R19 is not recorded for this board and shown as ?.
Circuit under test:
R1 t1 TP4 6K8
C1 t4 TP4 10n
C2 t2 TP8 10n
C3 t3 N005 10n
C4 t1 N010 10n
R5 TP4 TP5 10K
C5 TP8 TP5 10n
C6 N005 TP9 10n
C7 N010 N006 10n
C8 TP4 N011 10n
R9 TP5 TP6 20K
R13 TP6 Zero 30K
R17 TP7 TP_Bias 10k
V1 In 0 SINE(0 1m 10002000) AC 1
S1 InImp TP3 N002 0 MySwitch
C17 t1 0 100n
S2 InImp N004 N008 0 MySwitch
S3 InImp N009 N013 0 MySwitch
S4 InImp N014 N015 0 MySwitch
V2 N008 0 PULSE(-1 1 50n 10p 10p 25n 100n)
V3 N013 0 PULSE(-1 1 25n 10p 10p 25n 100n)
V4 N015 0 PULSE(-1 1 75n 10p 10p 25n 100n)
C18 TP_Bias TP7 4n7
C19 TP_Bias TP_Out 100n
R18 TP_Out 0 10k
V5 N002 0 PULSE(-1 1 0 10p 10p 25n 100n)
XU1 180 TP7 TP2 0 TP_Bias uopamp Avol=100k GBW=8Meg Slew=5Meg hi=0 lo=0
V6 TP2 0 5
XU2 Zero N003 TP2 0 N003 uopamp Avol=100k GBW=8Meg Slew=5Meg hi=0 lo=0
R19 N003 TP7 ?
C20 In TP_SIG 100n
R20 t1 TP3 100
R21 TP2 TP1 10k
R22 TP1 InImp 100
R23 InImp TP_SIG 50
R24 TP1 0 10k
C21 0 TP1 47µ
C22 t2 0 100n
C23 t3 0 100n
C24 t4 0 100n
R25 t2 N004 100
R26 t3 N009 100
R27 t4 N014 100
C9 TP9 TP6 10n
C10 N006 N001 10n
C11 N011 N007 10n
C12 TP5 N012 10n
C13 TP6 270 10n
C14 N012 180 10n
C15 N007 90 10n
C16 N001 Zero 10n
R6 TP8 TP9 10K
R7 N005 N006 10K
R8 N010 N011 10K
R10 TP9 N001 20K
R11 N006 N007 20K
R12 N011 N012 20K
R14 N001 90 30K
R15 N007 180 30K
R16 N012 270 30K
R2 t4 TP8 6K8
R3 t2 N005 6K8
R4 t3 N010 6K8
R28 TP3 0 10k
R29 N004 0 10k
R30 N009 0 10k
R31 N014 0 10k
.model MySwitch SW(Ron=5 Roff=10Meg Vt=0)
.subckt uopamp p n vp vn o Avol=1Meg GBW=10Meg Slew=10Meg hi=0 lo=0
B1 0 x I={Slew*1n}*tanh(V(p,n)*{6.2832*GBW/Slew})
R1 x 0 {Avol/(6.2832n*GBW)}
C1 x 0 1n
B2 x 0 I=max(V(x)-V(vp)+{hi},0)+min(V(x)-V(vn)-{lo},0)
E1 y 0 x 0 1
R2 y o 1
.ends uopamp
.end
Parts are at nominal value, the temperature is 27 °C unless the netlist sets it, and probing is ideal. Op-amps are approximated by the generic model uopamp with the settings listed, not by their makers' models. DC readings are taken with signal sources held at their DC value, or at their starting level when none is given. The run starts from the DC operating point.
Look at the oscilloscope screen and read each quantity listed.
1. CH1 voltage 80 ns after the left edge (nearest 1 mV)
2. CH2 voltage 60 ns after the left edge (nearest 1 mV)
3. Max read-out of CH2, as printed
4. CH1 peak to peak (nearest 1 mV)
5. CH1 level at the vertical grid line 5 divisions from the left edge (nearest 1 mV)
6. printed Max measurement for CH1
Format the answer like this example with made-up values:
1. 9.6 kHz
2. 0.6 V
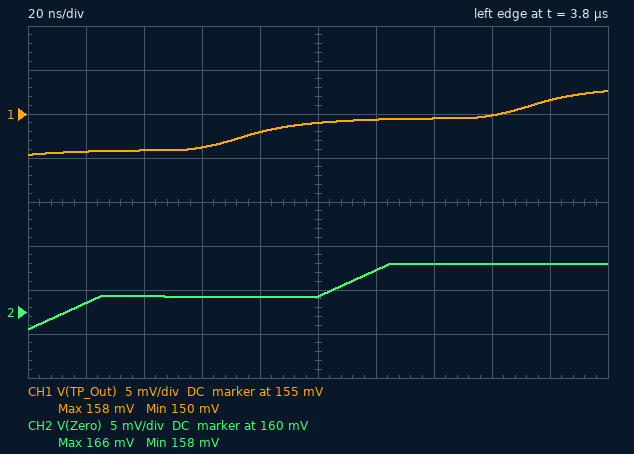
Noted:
1. 153 mV
2. 162 mV
3. 166 mV
4. 7 mV
5. 154 mV
6. 158 mV
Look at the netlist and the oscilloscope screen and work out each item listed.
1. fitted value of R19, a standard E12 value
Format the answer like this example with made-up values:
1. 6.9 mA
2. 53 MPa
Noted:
1. 330 Ω
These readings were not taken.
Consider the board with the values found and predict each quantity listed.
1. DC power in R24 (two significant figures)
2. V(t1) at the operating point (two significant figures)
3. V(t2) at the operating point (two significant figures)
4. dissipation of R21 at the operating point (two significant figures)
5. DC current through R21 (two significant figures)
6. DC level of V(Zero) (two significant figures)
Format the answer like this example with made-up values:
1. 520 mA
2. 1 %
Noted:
1. 620 µW
2. 2.5 mV
3. 2.5 mV
4. 630 µW
5. 250 µA
6. 2.5 mV
